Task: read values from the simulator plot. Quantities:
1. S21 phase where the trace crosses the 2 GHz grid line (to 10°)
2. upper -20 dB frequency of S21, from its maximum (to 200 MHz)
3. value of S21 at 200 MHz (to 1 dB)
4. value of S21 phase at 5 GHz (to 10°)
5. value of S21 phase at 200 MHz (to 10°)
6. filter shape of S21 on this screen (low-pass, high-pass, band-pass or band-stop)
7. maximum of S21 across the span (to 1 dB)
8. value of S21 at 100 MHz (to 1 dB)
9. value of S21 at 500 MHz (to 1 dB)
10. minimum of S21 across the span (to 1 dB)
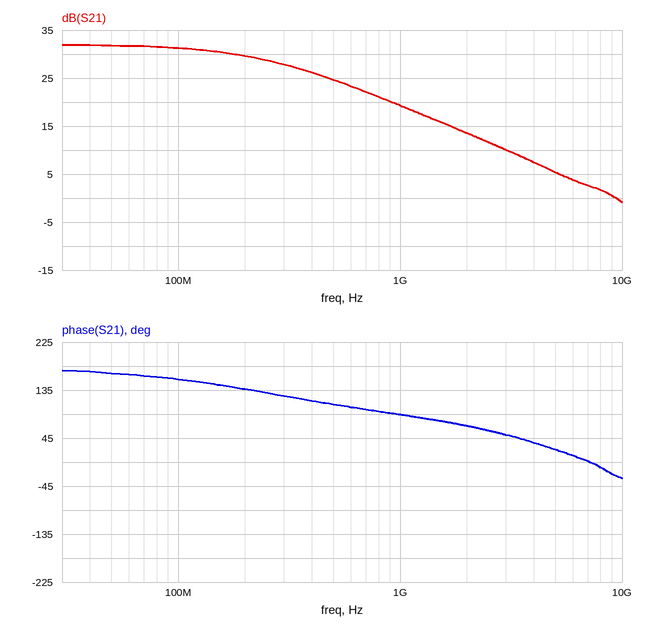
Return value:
70°
2.4 GHz
30 dB
20°
140°
low-pass
32 dB
31 dB
25 dB
-1 dB
